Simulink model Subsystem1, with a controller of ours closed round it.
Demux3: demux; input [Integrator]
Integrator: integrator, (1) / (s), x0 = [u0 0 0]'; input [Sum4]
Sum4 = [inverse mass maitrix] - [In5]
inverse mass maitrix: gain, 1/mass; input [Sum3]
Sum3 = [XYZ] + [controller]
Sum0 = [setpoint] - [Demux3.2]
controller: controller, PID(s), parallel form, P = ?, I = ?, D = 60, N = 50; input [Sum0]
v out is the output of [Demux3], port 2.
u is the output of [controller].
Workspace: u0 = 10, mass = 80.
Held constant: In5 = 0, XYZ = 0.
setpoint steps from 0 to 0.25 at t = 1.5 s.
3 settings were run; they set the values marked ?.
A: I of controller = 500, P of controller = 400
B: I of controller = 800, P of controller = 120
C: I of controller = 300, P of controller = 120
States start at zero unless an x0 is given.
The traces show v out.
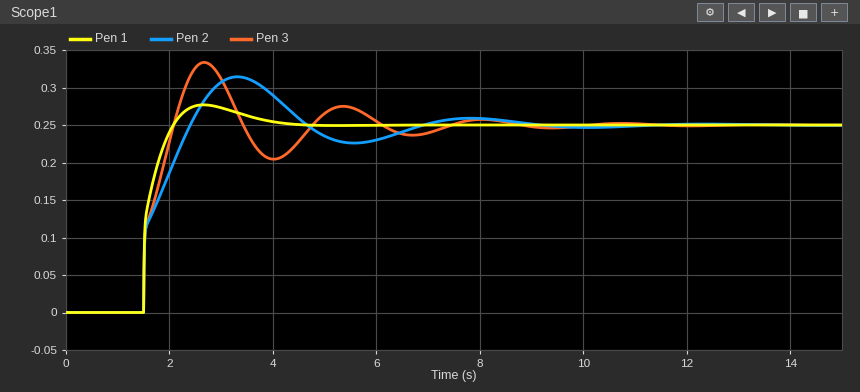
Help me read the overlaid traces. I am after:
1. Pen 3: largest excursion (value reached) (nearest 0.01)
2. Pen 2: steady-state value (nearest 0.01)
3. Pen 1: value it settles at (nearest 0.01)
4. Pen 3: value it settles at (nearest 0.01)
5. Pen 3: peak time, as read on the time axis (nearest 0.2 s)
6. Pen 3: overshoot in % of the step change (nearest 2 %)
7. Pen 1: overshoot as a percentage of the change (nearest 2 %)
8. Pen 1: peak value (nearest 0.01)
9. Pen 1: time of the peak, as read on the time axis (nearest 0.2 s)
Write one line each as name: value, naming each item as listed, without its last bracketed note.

Pen 3: largest excursion (value reached): 0.33
Pen 2: steady-state value: 0.25
Pen 1: value it settles at: 0.25
Pen 3: value it settles at: 0.25
Pen 3: peak time, as read on the time axis: 2.6 s
Pen 3: overshoot in % of the step change: 34 %
Pen 1: overshoot as a percentage of the change: 10 %
Pen 1: peak value: 0.28
Pen 1: time of the peak, as read on the time axis: 2.6 s
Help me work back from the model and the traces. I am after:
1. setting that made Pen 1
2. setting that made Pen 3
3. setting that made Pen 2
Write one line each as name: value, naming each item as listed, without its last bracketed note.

setting that made Pen 1: A
setting that made Pen 3: B
setting that made Pen 2: C
